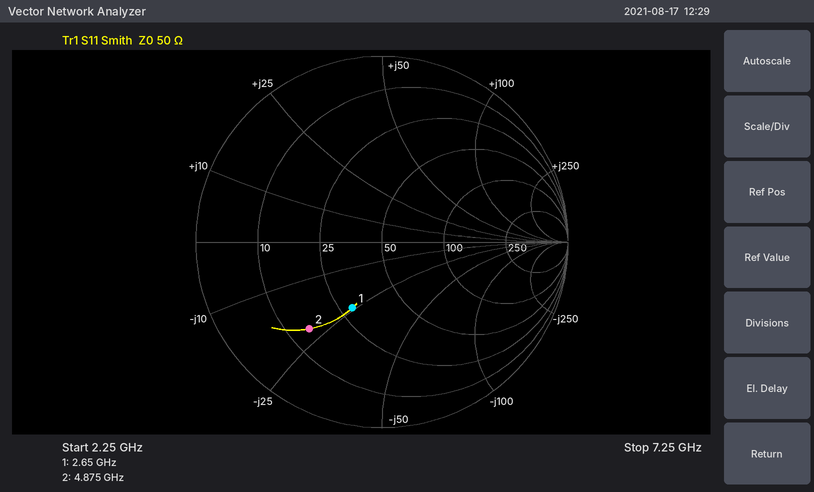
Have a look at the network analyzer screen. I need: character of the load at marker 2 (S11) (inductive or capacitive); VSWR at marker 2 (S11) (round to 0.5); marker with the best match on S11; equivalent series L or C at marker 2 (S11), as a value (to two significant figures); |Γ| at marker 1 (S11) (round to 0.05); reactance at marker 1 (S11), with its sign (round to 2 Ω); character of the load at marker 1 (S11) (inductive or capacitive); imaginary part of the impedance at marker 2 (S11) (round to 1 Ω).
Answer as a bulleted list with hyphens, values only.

- capacitive
- 4.0
- marker 1
- 1.5 pF
- 0.40
- -24 Ω
- capacitive
- -22 Ω
